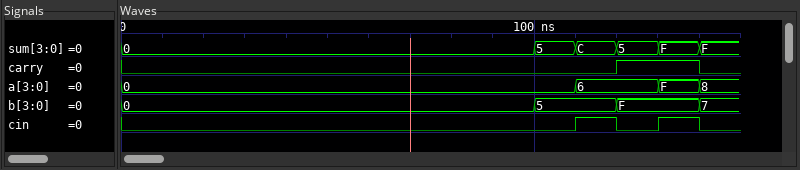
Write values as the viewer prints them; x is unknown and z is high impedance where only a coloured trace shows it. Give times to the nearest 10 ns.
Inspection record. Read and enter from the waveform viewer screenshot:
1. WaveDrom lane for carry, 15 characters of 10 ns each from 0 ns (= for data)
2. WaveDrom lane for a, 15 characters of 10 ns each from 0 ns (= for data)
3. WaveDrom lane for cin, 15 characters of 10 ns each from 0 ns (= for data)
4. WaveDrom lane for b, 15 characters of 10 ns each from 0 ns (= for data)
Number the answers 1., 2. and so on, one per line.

1. {name: 'carry', wave: '0...........1.0'}
2. {name: 'a', wave: '=..........=.==', data: '0 6 F 8'}
3. {name: 'cin', wave: '0..........1010'}
4. {name: 'b', wave: '=.........=.=.=', data: '0 5 F 7'}
